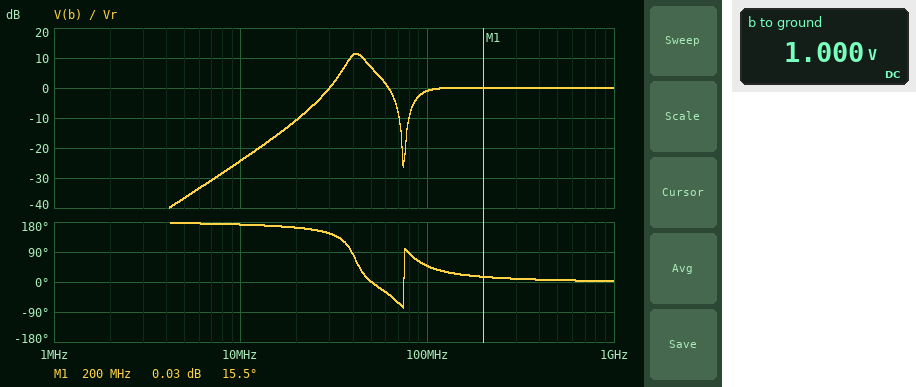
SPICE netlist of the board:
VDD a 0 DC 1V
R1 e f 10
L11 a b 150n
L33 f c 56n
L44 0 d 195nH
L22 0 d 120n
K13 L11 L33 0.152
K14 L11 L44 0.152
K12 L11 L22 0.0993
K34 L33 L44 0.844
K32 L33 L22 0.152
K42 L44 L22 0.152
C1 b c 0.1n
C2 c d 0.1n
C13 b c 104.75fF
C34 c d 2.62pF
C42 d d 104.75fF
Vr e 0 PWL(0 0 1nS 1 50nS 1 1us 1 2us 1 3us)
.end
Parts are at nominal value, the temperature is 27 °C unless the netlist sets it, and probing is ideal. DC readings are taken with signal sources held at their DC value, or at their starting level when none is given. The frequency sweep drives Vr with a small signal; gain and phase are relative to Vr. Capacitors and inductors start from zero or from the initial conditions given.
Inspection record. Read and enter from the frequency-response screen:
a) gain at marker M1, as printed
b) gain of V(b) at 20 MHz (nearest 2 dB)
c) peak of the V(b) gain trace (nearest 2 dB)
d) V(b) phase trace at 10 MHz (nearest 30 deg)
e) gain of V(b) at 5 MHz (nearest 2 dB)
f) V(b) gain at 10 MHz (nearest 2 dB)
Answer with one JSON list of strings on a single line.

["0.03 dB", "-10 dB", "12 dB", "180 deg", "-36 dB", "-24 dB"]
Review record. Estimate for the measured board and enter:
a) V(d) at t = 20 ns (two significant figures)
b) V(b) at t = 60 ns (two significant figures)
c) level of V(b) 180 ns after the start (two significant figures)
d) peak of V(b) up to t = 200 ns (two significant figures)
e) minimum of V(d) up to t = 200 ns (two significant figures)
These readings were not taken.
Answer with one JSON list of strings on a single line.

["-82 mV", "1.0 V", "1.0 V", "1.4 V", "-650 mV"]
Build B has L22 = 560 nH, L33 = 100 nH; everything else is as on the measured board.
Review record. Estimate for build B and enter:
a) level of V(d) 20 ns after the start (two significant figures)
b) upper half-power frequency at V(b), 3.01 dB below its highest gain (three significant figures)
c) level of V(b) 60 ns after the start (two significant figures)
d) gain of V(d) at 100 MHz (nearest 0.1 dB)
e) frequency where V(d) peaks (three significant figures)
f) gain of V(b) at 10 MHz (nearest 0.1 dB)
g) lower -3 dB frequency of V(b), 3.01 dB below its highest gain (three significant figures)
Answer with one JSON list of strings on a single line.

["130 mV", "41.1 MHz", "1.1 V", "3.5 dB", "65.8 MHz", "-24.6 dB", "33.6 MHz"]
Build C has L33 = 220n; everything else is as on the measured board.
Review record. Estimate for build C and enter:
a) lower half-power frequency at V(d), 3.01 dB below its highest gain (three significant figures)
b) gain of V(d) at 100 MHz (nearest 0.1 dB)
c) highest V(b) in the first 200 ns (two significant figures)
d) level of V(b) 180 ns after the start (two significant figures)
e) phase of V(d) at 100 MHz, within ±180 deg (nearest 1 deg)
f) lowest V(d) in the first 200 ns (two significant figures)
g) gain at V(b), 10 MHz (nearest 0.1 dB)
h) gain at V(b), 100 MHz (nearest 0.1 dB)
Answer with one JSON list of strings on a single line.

["60.4 MHz", "-9.6 dB", "1.7 V", "1.0 V", "23 deg", "-390 mV", "-25.0 dB", "-7.8 dB"]
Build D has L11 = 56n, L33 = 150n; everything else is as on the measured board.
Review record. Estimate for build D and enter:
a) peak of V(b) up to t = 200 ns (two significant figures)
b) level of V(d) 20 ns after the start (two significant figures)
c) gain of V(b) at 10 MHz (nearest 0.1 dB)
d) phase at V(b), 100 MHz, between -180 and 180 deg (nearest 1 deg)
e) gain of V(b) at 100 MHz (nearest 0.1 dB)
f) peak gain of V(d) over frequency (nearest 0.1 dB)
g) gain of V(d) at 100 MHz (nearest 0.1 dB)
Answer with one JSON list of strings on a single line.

["1.3 V", "-400 mV", "-34.3 dB", "-145 deg", "-20.0 dB", "9.7 dB", "-0.7 dB"]
